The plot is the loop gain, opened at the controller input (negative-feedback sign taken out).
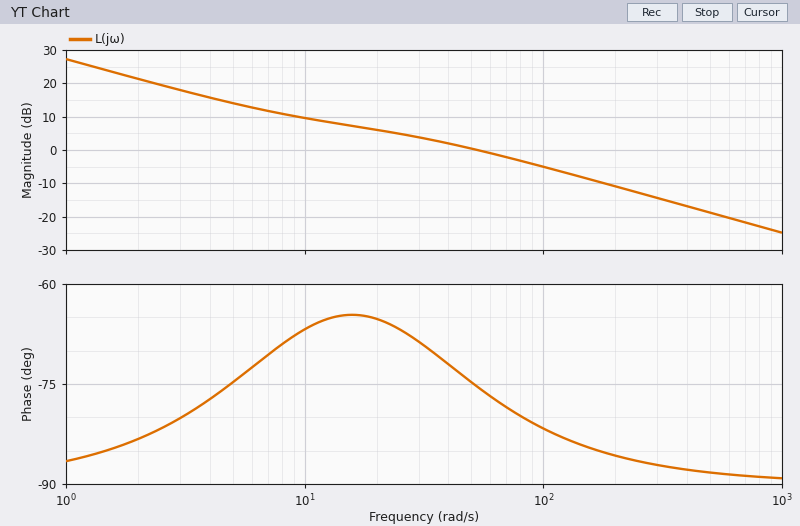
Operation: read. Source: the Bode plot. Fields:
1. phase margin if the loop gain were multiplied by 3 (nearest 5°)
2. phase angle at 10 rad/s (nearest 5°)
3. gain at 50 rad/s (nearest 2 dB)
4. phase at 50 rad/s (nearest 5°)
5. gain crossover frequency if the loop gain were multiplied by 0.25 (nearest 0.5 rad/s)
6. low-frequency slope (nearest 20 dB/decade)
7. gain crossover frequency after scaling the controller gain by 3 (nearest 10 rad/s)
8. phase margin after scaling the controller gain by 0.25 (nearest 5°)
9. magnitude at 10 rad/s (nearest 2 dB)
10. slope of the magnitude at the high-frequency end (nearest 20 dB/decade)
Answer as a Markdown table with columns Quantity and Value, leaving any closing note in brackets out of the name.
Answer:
| Quantity | Value |
|---|---|
| phase margin if the loop gain were multiplied by 3 | 95° |
| phase angle at 10 rad/s | -65° |
| gain at 50 rad/s | 0 dB |
| phase at 50 rad/s | -75° |
| gain crossover frequency if the loop gain were multiplied by 0.25 | 6.5 rad/s |
| low-frequency slope | -20 dB/decade |
| gain crossover frequency after scaling the controller gain by 3 | 170 rad/s |
| phase margin after scaling the controller gain by 0.25 | 110° |
| magnitude at 10 rad/s | 10 dB |
| slope of the magnitude at the high-frequency end | -20 dB/decade |
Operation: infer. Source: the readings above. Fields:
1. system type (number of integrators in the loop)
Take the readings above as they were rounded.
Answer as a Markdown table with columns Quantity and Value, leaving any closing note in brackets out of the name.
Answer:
| Quantity | Value |
|---|---|
| system type | 1 |
